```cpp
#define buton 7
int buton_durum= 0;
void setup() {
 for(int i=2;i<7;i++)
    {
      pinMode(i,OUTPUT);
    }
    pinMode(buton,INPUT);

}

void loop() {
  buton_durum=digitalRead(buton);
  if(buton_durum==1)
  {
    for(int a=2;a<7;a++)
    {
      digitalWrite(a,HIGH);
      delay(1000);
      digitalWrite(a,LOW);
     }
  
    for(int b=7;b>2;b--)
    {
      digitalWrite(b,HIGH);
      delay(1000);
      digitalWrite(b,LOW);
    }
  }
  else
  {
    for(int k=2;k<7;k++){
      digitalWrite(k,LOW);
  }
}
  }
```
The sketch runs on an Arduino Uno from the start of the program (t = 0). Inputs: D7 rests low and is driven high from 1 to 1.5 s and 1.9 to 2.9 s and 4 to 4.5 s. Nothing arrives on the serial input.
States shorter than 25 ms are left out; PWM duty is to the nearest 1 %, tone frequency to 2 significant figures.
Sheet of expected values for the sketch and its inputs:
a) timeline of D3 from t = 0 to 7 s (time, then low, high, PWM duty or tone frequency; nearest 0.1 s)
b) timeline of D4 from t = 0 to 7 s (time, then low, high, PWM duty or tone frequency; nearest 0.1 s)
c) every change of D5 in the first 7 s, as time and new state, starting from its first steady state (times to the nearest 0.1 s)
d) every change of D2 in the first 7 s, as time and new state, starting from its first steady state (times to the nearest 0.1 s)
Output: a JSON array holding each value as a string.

["0 s low; 2 s high; 3 s low", "0 s low; 3 s high; 4 s low", "0 s low; 4 s high; 5 s low", "0 s low; 1 s high; 2 s low"]
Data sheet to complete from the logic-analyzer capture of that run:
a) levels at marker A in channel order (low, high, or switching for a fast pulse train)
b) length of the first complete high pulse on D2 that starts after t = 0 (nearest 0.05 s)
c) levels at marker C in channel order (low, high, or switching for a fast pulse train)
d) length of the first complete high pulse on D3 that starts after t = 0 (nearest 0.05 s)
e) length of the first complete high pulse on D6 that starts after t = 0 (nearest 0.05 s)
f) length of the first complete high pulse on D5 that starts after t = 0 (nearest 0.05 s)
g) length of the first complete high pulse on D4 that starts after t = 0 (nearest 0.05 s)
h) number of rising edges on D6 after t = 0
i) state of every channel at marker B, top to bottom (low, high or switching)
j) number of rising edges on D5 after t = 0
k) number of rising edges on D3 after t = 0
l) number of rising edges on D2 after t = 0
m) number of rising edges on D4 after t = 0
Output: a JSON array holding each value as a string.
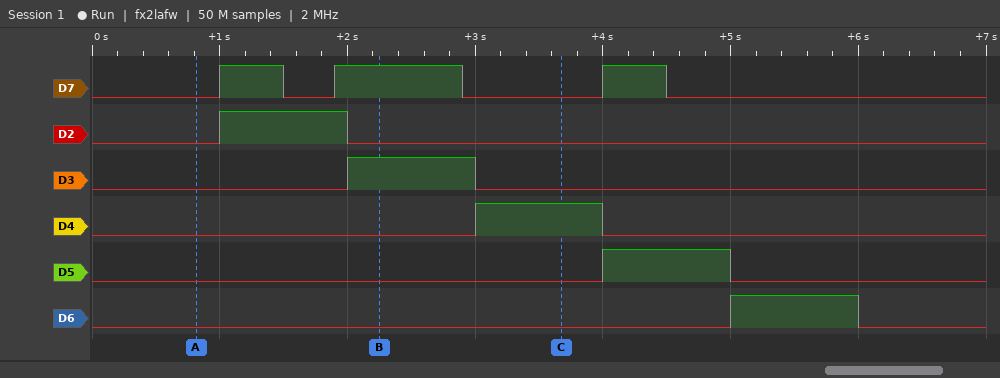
["D7 low, D2 low, D3 low, D4 low, D5 low, D6 low", "1.00 s", "D7 low, D2 low, D3 low, D4 high, D5 low, D6 low", "1.00 s", "1.00 s", "1.00 s", "1.00 s", "1", "D7 high, D2 low, D3 high, D4 low, D5 low, D6 low", "1", "1", "1", "1"]
